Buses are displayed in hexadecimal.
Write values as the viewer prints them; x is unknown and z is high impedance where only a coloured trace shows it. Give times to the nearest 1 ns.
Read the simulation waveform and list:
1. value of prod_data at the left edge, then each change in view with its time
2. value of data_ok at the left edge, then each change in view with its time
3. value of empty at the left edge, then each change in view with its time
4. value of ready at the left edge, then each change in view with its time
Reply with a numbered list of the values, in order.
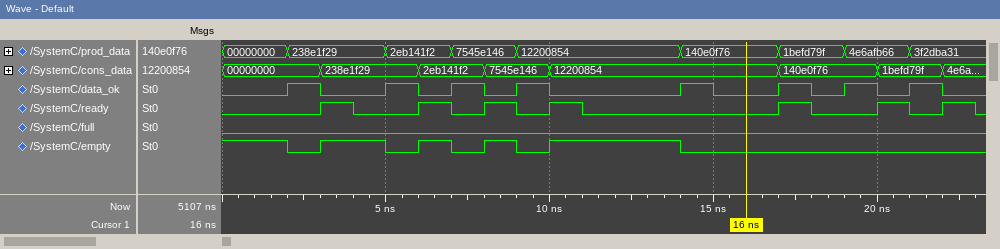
1. 00000000, 238e1f29 at 2 ns, 2eb141f2 at 5 ns, 7545e146 at 7 ns, 12200854 at 9 ns, 140e0f76 at 14 ns, 1befd79f at 17 ns, 4e6afb66 at 19 ns, 3f2dba31 at 21 ns
2. 0, 1 at 2 ns, 0 at 3 ns, 1 at 5 ns, 0 at 6 ns, 1 at 7 ns, 0 at 8 ns, 1 at 9 ns, 0 at 10 ns, 1 at 14 ns, 0 at 15 ns, 1 at 17 ns, 0 at 18 ns, 1 at 19 ns, 0 at 20 ns, 1 at 21 ns, 0 at 22 ns
3. 1, 0 at 2 ns, 1 at 3 ns, 0 at 5 ns, 1 at 6 ns, 0 at 7 ns, 1 at 8 ns, 0 at 9 ns, 1 at 10 ns, 0 at 14 ns
4. 0, 1 at 3 ns, 0 at 4 ns, 1 at 6 ns, 0 at 7 ns, 1 at 8 ns, 0 at 9 ns, 1 at 10 ns, 0 at 11 ns, 1 at 17 ns, 0 at 18 ns, 1 at 20 ns, 0 at 21 ns, 1 at 22 ns, 0 at 23 ns
